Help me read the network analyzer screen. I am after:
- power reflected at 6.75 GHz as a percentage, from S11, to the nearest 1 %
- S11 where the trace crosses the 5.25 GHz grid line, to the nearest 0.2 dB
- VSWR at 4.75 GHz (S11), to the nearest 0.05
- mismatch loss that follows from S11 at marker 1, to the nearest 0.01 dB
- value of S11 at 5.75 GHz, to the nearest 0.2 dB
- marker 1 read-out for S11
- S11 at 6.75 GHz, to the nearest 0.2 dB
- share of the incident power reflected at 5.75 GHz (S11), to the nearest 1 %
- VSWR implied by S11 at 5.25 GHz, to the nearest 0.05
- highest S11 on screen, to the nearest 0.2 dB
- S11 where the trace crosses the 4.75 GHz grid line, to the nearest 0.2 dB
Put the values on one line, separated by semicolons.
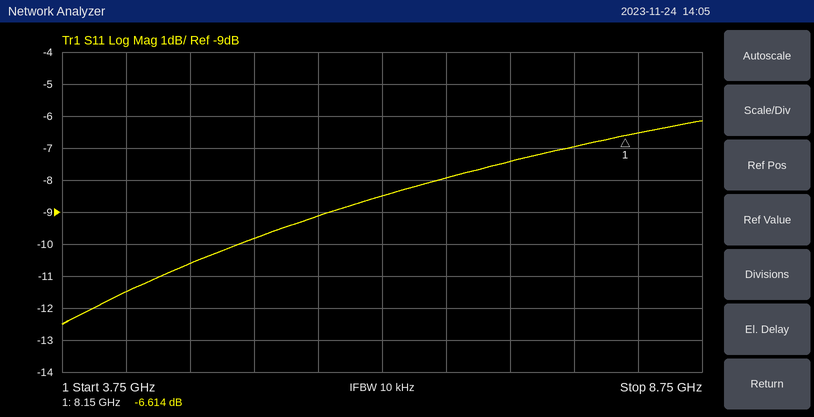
16 %; -9.8 dB; 1.85; 1.07 dB; -9.2 dB; -6.614 dB; -8.0 dB; 12 %; 1.95; -6.2 dB; -10.6 dB
